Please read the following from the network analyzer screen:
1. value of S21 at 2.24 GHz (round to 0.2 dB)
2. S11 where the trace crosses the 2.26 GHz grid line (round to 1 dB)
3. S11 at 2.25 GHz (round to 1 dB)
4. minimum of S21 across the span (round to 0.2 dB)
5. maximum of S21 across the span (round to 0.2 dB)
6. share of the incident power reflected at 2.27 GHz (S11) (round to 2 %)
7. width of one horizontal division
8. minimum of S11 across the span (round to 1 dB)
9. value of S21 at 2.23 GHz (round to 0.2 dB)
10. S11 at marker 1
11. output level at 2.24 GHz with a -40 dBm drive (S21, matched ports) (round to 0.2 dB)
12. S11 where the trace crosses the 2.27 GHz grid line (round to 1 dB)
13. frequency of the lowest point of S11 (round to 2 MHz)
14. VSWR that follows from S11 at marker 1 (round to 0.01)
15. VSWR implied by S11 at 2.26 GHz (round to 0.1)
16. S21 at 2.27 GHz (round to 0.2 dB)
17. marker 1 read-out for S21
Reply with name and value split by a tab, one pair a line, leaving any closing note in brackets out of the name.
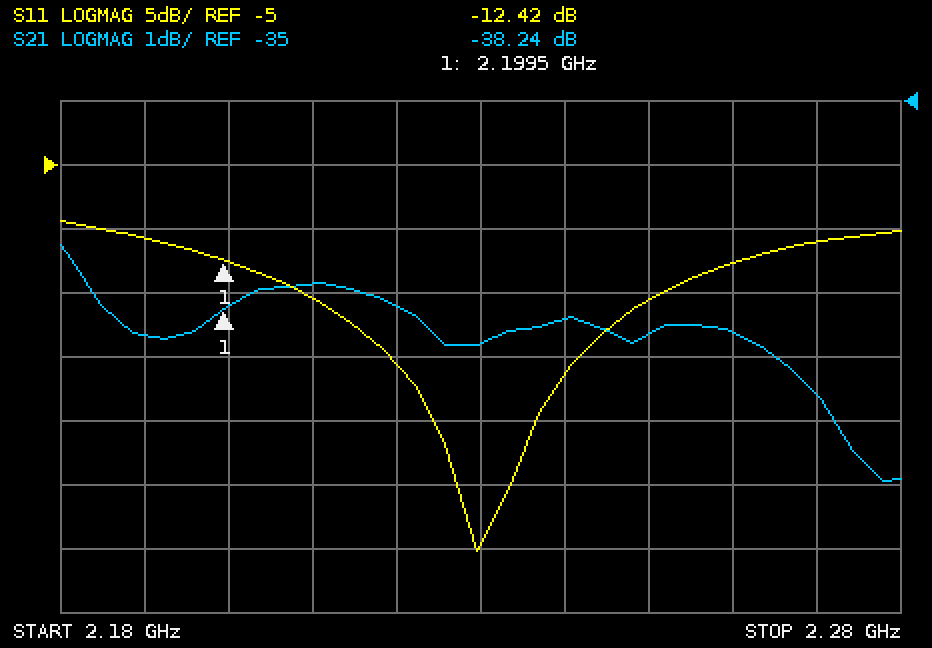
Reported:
value of S21 at 2.24 GHz	-38.4 dB
S11 where the trace crosses the 2.26 GHz grid line	-13 dB
S11 at 2.25 GHz	-16 dB
minimum of S21 across the span	-41.0 dB
maximum of S21 across the span	-37.2 dB
share of the incident power reflected at 2.27 GHz (S11)	8 %
width of one horizontal division	10 MHz
minimum of S11 across the span	-35 dB
value of S21 at 2.23 GHz	-38.8 dB
S11 at marker 1	-12.42 dB
output level at 2.24 GHz with a -40 dBm drive (S21, matched ports)	-78.4 dBm
S11 where the trace crosses the 2.27 GHz grid line	-11 dB
frequency of the lowest point of S11	2.230 GHz
VSWR that follows from S11 at marker 1	1.63
VSWR implied by S11 at 2.26 GHz	1.6
S21 at 2.27 GHz	-39.6 dB
marker 1 read-out for S21	-38.24 dB
